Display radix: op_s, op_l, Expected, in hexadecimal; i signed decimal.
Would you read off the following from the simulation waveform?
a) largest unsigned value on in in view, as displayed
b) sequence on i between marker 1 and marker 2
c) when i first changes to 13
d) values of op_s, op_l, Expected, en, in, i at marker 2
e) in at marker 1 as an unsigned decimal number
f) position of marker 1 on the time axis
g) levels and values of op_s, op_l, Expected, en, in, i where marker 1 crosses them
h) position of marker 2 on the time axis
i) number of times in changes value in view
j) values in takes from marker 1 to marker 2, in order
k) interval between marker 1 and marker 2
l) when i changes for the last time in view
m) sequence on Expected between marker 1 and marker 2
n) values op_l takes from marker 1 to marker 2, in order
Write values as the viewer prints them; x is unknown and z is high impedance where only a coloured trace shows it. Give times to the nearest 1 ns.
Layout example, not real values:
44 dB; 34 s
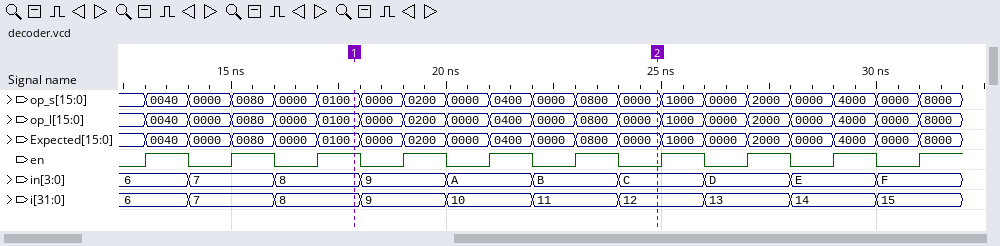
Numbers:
F; 8, 9, 10, 11, 12; 26 ns; op_s=0000, op_l=0000, Expected=0000, en=0, in=C, i=12; 8; 18 ns; op_s=0100, op_l=0100, Expected=0100, en=1, in=8, i=8; 25 ns; 9; 8, 9, A, B, C; 7 ns; 30 ns; 0100, 0000, 0200, 0000, 0400, 0000, 0800, 0000; 0100, 0000, 0200, 0000, 0400, 0000, 0800, 0000
